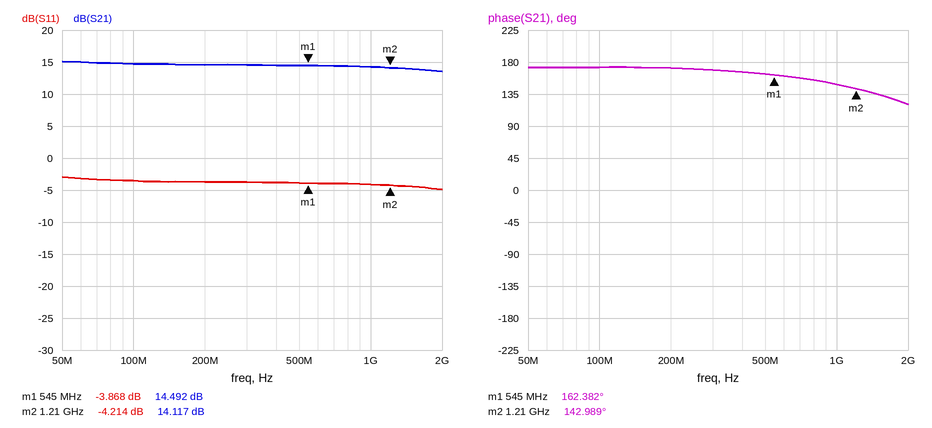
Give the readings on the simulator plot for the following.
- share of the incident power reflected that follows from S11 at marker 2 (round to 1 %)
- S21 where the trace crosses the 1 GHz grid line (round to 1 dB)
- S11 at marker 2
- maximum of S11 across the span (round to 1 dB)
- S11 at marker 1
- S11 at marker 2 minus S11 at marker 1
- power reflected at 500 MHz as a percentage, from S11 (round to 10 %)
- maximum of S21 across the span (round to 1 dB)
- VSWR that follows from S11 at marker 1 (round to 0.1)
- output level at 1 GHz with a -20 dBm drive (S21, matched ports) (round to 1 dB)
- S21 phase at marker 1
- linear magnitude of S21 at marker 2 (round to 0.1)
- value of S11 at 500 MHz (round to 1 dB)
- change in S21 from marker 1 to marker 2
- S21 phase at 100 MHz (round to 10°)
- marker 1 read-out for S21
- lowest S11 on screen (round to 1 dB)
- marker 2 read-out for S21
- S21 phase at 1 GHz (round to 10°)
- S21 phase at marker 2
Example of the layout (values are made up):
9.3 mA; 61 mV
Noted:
38 %; 14 dB; -4.214 dB; -3 dB; -3.868 dB; -0.346 dB; 40 %; 15 dB; 4.6; -6 dBm; 162.382°; 5.1; -4 dB; -0.375 dB; 170°; 14.492 dB; -5 dB; 14.117 dB; 150°; 142.989°
